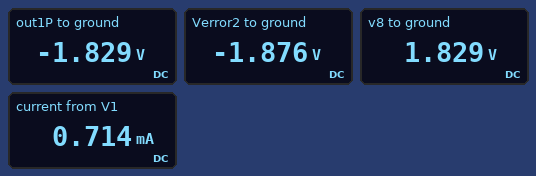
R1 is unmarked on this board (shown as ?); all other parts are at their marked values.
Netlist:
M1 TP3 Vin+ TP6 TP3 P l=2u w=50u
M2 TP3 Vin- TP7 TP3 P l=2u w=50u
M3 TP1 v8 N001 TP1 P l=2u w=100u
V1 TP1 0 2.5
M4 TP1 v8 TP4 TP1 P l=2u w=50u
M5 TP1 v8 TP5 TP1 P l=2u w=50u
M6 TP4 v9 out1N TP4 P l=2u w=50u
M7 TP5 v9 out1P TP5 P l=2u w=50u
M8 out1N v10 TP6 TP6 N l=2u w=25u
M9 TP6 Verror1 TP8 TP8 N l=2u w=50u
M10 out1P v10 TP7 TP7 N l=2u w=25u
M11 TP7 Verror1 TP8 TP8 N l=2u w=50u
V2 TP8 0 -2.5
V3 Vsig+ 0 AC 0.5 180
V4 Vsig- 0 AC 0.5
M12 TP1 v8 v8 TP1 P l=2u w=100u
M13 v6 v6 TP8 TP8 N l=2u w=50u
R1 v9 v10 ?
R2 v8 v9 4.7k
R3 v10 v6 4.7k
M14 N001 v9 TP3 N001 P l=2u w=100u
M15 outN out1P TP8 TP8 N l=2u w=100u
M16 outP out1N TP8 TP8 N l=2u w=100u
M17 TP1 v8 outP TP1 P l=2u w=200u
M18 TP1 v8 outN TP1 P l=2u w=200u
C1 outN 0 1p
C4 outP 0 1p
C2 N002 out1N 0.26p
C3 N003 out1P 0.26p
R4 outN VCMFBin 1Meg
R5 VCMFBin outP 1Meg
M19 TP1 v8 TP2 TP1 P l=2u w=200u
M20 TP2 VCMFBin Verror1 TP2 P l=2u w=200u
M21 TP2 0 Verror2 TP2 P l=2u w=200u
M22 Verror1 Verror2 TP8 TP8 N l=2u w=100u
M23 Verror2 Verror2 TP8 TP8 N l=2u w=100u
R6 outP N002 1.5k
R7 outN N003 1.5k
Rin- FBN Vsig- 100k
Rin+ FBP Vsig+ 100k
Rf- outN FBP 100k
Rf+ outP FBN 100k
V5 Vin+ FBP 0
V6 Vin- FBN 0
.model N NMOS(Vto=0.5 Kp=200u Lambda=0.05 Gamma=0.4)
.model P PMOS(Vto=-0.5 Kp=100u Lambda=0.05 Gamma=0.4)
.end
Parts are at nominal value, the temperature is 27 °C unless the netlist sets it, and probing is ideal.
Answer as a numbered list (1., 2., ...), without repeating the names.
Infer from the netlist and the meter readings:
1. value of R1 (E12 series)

1. 39 kΩ
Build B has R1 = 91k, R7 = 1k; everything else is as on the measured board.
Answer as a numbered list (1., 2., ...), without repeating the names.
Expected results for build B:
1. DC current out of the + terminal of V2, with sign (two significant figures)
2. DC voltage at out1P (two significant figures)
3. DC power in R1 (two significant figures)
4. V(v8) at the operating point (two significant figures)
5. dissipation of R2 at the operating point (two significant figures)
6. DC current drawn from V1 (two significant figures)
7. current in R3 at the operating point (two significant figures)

1. -350 µA
2. -1.9 V
3. 130 µW
4. 1.9 V
5. 6.6 µW
6. 350 µA
7. 37 µA
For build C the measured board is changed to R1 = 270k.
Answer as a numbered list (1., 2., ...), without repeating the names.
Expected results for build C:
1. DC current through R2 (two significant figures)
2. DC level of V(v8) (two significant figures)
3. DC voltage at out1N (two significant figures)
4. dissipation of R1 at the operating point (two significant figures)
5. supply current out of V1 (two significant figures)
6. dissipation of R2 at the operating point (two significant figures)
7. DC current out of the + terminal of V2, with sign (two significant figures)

1. 14 µA
2. 1.9 V
3. -1.9 V
4. 51 µW
5. 130 µA
6. 890 nW
7. -130 µA
